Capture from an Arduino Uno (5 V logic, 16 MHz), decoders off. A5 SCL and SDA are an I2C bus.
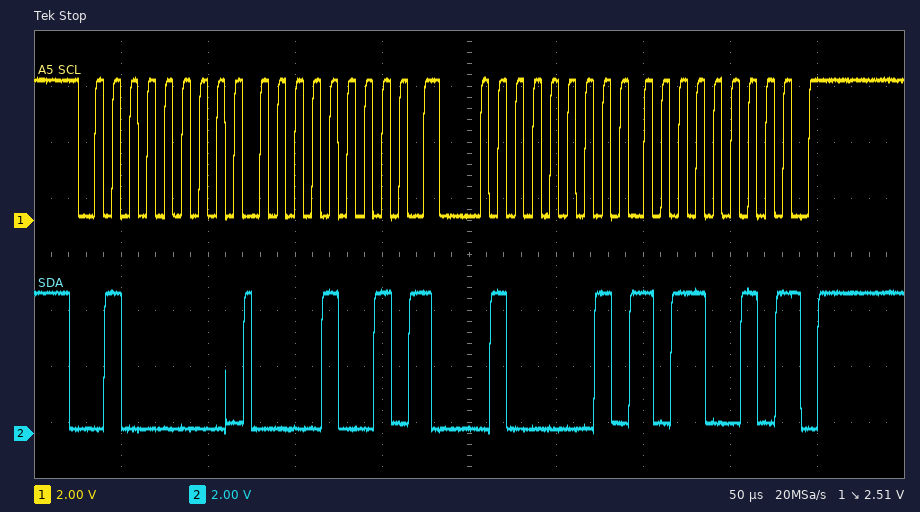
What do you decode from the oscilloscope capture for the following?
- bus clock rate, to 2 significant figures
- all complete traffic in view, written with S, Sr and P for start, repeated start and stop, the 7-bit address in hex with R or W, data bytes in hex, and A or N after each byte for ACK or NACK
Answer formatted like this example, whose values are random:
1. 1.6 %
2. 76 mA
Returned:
1. 100 kHz
2. S 20W A 09 A Sr 20R A B2 N P
